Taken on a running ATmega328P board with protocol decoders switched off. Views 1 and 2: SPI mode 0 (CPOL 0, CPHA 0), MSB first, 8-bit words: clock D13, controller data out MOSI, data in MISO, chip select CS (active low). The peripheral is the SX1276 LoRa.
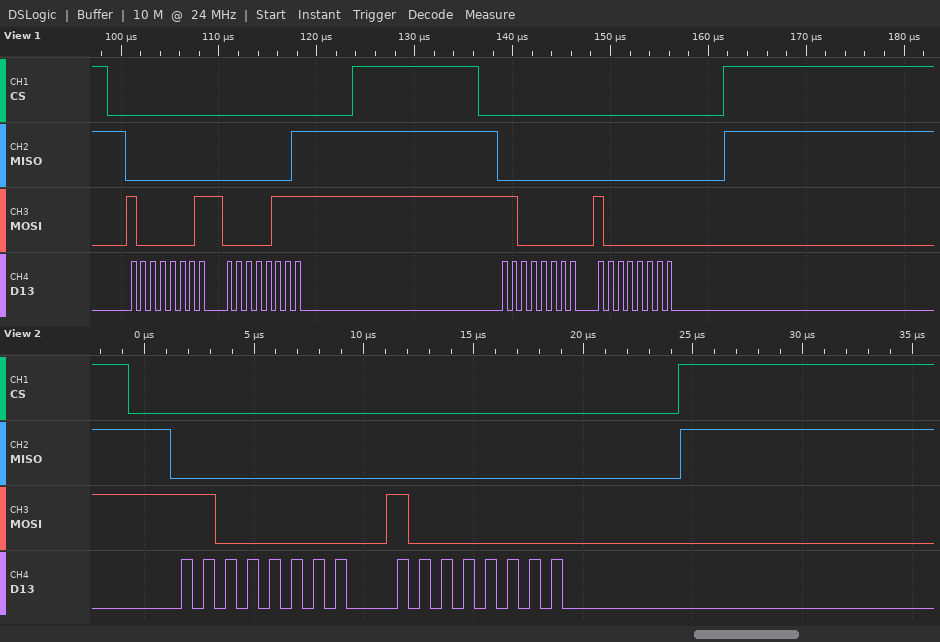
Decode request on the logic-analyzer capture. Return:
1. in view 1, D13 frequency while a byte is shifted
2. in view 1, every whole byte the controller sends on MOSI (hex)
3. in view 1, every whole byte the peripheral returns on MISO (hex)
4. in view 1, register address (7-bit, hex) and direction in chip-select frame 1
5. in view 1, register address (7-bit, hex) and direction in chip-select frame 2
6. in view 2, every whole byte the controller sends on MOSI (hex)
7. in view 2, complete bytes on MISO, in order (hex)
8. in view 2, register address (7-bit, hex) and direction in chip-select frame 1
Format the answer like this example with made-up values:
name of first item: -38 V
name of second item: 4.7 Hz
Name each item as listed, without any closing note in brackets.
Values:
in view 1, D13 frequency while a byte is shifted: 1 MHz
in view 1, every whole byte the controller sends on MOSI: 81 07 C0 80
in view 1, every whole byte the peripheral returns on MISO: 00 01 00 00
in view 1, register address (7-bit, hex) and direction in chip-select frame 1: 0x01 write
in view 1, register address (7-bit, hex) and direction in chip-select frame 2: 0x40 write
in view 2, every whole byte the controller sends on MOSI: 0xC0 0x80
in view 2, complete bytes on MISO, in order: 0x00 0x00
in view 2, register address (7-bit, hex) and direction in chip-select frame 1: 0x40 write
